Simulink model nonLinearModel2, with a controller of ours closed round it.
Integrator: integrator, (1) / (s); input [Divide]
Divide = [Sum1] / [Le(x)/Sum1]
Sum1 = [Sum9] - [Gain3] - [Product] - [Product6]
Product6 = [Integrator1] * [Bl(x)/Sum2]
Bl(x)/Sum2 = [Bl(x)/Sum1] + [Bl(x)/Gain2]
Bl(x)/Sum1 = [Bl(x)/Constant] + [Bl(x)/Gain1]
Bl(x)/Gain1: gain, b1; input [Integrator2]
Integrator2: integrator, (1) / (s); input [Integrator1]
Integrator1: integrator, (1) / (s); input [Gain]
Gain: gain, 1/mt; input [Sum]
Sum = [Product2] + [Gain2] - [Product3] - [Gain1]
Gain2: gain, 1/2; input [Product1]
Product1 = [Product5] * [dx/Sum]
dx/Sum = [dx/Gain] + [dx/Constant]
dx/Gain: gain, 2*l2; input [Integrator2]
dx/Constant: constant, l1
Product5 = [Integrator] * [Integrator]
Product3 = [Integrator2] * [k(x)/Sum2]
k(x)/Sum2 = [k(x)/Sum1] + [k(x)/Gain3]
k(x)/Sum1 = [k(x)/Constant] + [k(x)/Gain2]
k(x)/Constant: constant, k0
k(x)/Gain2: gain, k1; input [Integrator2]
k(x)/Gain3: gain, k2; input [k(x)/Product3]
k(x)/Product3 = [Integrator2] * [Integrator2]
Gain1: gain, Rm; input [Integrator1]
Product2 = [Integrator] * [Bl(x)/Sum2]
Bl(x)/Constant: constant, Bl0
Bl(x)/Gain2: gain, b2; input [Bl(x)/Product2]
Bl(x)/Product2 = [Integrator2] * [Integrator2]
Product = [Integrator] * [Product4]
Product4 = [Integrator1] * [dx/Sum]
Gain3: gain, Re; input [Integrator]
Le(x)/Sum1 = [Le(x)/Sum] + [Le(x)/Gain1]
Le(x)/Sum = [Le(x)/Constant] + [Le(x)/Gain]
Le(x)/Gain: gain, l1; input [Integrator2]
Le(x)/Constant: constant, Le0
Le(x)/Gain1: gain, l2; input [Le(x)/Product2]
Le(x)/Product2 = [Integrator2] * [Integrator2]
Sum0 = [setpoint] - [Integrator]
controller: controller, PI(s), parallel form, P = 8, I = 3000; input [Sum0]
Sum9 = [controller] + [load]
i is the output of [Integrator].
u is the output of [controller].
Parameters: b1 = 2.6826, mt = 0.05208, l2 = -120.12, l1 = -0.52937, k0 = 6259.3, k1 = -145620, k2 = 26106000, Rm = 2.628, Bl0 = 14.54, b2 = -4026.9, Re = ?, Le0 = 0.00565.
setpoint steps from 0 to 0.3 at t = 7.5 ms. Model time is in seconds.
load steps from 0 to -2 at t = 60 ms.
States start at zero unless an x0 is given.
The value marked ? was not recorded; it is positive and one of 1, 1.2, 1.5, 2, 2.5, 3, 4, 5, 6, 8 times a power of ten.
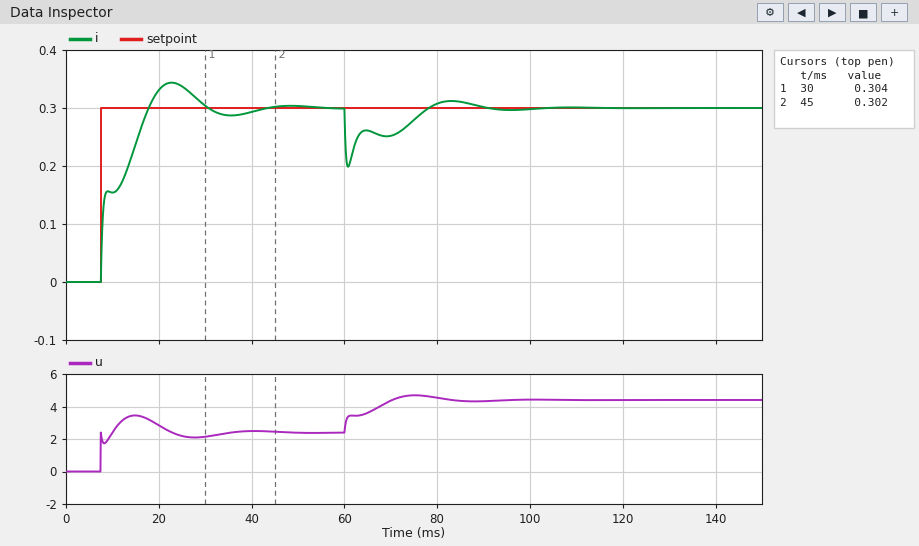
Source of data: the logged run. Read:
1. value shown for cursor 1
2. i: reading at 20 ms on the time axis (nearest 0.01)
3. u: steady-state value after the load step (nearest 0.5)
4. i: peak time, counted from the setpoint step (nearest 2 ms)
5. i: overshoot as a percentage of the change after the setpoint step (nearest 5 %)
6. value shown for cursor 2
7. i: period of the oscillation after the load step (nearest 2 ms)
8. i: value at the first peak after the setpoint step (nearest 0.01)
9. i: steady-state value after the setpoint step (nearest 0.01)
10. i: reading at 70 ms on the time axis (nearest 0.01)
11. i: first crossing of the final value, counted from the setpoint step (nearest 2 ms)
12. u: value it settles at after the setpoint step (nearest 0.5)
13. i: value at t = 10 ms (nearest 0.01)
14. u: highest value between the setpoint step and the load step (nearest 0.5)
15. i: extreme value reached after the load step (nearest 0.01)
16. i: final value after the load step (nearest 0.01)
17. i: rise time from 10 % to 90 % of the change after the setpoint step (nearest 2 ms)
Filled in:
0.304
0.33
4.5
16 ms
15 %
0.302
8 ms
0.34
0.30
0.25
10 ms
2.5
0.15
3.5
0.20
0.30
8 ms
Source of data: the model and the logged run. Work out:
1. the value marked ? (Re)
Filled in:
8
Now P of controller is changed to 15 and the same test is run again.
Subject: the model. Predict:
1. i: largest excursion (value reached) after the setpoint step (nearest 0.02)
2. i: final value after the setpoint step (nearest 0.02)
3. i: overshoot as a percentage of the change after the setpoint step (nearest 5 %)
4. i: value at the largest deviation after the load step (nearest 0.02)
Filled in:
0.32
0.30
10 %
0.22
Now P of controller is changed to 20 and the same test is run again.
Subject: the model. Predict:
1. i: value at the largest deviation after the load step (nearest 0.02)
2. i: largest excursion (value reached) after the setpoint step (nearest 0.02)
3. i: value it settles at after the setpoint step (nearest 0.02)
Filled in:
0.24
0.32
0.30
